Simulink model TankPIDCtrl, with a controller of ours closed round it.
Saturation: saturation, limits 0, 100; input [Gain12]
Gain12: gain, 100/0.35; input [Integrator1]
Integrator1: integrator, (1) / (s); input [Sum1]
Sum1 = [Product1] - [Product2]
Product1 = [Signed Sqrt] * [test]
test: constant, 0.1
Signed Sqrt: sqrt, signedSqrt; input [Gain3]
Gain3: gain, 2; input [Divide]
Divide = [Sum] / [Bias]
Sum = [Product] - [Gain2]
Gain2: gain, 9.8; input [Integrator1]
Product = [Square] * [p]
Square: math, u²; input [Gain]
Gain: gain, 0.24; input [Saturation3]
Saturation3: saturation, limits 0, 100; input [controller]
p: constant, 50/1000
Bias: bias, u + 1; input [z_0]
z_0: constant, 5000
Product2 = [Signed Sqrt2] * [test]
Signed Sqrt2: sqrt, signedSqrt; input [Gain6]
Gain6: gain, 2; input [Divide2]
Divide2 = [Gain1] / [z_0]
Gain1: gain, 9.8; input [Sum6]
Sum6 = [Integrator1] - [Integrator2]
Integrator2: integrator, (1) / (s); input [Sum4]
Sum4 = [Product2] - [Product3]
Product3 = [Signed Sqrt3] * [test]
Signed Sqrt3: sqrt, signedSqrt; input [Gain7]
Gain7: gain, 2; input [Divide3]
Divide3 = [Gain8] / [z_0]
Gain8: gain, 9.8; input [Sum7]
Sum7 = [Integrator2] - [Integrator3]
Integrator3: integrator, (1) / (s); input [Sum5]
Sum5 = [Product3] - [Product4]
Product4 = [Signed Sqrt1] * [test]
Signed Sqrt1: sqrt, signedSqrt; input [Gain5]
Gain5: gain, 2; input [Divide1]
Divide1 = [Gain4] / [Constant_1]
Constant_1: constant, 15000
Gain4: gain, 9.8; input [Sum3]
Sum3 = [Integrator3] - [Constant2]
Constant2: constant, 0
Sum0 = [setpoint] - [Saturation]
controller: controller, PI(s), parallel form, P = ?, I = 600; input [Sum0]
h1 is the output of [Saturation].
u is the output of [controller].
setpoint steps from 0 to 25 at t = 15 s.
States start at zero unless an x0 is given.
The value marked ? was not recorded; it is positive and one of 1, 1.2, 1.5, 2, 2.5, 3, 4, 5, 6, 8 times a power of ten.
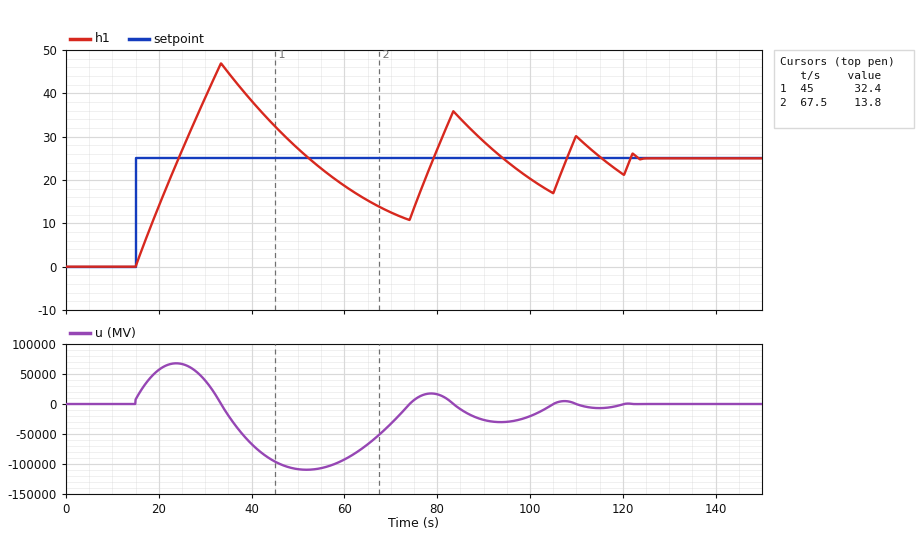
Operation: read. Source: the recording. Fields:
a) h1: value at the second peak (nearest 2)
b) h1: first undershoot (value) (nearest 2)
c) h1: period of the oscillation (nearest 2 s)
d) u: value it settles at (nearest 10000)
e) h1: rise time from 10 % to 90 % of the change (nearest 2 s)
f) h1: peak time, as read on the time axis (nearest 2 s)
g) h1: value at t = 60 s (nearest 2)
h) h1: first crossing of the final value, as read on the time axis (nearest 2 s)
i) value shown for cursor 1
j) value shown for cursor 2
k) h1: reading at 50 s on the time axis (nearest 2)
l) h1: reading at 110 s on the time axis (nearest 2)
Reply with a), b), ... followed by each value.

a) 36
b) 10
c) 50 s
d) 0
e) 8 s
f) 34 s
g) 18
h) 24 s
i) 32.4
j) 13.8
k) 28
l) 30
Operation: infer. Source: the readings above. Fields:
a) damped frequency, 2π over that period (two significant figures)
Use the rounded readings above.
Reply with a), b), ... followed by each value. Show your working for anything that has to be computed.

a) 2π / 50 = 0.13 rad/s
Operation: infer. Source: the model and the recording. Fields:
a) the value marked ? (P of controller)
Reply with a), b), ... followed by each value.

a) 300
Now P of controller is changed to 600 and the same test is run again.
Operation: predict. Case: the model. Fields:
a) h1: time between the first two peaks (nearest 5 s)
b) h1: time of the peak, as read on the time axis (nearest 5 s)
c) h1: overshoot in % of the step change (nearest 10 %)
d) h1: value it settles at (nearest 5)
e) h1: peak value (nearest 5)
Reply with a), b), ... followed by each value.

a) 45 s
b) 35 s
c) 80 %
d) 25
e) 45
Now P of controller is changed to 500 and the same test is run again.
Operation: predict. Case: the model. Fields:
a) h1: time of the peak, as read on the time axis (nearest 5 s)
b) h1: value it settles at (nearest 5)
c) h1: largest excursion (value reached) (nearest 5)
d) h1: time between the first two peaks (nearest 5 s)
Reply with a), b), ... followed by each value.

a) 35 s
b) 25
c) 45
d) 45 s
